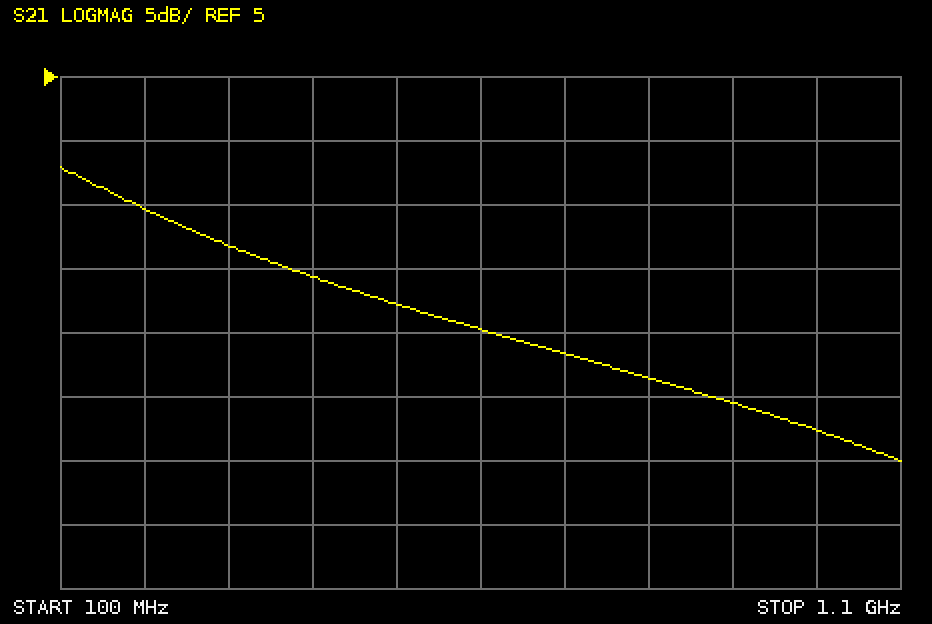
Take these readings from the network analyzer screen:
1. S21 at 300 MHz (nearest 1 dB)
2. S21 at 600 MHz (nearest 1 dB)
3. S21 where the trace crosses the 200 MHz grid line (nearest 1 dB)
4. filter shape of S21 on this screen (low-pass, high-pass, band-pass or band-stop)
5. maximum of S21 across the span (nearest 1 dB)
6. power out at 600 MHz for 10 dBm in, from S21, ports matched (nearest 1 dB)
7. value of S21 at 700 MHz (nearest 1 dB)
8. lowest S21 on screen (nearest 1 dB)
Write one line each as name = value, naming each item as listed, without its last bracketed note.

S21 at 300 MHz = -8 dB
S21 at 600 MHz = -15 dB
S21 where the trace crosses the 200 MHz grid line = -5 dB
filter shape of S21 on this screen = low-pass
maximum of S21 across the span = -2 dB
power out at 600 MHz for 10 dBm in, from S21, ports matched = -5 dBm
value of S21 at 700 MHz = -17 dB
lowest S21 on screen = -25 dB
